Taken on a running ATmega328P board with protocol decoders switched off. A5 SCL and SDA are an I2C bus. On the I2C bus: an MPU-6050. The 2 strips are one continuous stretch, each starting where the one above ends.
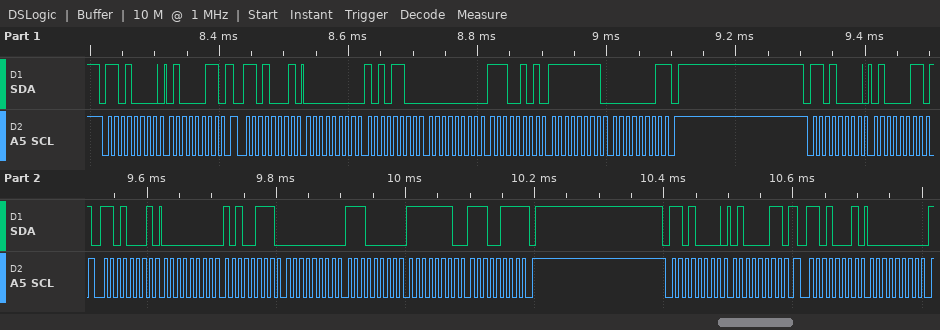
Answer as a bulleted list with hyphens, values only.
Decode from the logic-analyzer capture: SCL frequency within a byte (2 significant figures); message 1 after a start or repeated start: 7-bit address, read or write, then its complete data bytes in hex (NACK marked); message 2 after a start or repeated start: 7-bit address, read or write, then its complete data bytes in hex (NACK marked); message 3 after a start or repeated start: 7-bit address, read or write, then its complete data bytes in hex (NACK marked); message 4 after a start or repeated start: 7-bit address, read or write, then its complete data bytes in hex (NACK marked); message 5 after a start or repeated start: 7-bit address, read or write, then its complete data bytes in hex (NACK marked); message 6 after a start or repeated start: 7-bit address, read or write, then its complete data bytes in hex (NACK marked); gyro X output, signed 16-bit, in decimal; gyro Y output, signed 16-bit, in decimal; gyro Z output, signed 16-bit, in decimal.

- 100 kHz
- 0x68 write: 43
- 0x68 read: 00 AC 00 E5 FF 01 NACK
- 0x68 write: 43
- 0x68 read: 00 A7 00 E0 FE E7 NACK
- 0x68 write: 43
- 0x68 read: 00
- 172
- 229
- -255
